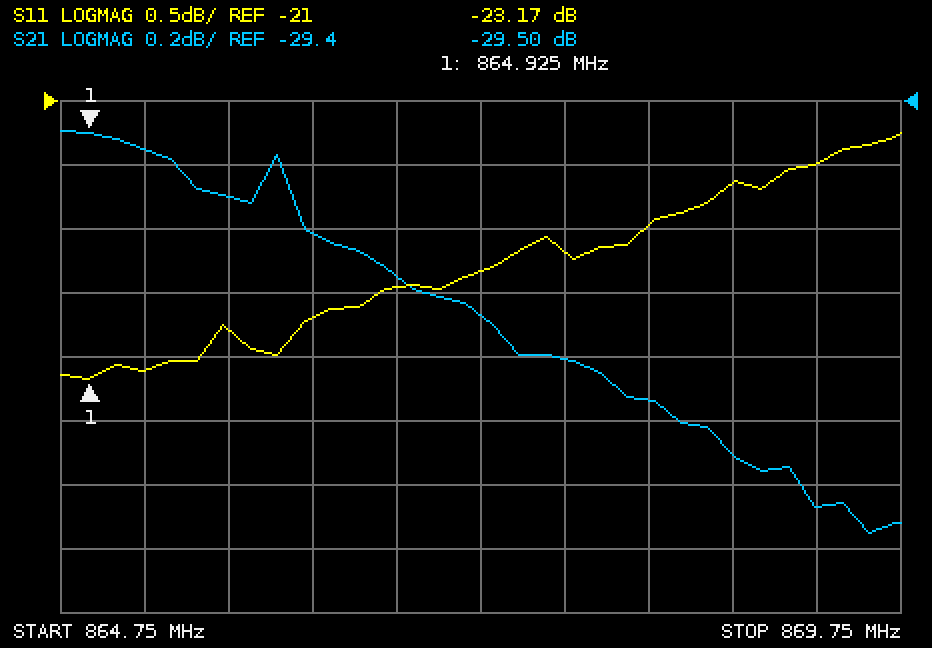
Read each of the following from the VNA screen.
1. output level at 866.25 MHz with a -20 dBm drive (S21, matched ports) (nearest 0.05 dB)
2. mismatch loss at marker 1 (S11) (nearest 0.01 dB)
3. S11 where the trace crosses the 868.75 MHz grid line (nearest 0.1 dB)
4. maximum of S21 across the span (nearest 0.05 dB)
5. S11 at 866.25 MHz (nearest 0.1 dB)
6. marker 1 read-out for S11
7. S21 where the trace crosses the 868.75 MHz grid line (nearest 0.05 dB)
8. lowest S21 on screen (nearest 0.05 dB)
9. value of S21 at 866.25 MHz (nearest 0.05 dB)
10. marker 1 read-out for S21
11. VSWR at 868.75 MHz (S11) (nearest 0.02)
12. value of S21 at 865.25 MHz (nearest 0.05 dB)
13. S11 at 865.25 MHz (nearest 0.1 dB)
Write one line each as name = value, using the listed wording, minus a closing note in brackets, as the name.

output level at 866.25 MHz with a -20 dBm drive (S21, matched ports) = -49.80 dBm
mismatch loss at marker 1 (S11) = 0.02 dB
S11 where the trace crosses the 868.75 MHz grid line = -21.6 dB
maximum of S21 across the span = -29.50 dB
S11 at 866.25 MHz = -22.7 dB
marker 1 read-out for S11 = -23.17 dB
S21 where the trace crosses the 868.75 MHz grid line = -30.50 dB
lowest S21 on screen = -30.75 dB
value of S21 at 866.25 MHz = -29.80 dB
marker 1 read-out for S21 = -29.50 dB
VSWR at 868.75 MHz (S11) = 1.18
value of S21 at 865.25 MHz = -29.55 dB
S11 at 865.25 MHz = -23.1 dB
